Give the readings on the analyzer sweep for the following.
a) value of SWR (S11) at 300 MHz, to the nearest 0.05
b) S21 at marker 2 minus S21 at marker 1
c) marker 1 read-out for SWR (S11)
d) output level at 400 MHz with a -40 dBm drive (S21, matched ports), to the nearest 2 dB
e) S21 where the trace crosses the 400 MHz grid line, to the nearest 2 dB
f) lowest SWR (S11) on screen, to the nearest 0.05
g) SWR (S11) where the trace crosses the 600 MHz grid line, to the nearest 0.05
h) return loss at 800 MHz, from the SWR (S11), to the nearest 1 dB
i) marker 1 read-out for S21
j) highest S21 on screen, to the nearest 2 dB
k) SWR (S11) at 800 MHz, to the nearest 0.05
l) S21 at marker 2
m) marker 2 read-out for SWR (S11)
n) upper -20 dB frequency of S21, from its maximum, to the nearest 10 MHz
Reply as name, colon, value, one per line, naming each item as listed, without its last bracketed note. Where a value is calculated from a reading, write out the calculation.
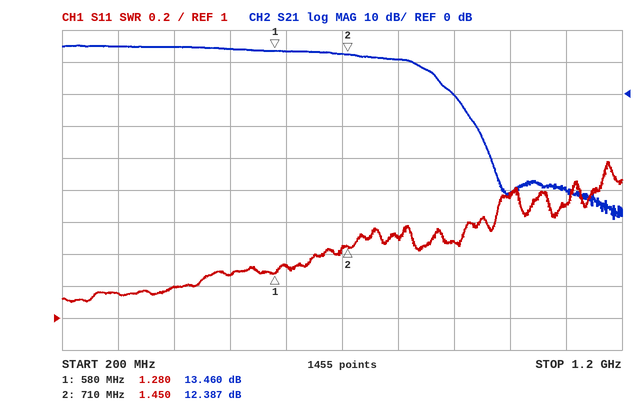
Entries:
value of SWR (S11) at 300 MHz, to the nearest 0.05: 1.15
S21 at marker 2 minus S21 at marker 1: 12.387 − (13.46) = -1.073 dB
marker 1 read-out for SWR: 1.280
output level at 400 MHz with a -40 dBm drive (S21, matched ports), to the nearest 2 dB: -40 dBm + (14 dB) = -26 dBm
S21 where the trace crosses the 400 MHz grid line, to the nearest 2 dB: 14 dB
lowest SWR (S11) on screen, to the nearest 0.05: 1.10
SWR (S11) where the trace crosses the 600 MHz grid line, to the nearest 0.05: 1.35
return loss at 800 MHz, from the SWR (S11), to the nearest 1 dB: −20 log10((1.5 − 1)/(1.5 + 1)) ≈ 14 dB
marker 1 read-out for S21: 13.460 dB
highest S21 on screen, to the nearest 2 dB: 16 dB
SWR (S11) at 800 MHz, to the nearest 0.05: 1.50
S21 at marker 2: 12.387 dB
marker 2 read-out for SWR: 1.450
upper -20 dB frequency of S21, from its maximum, to the nearest 10 MHz: 920 MHz
